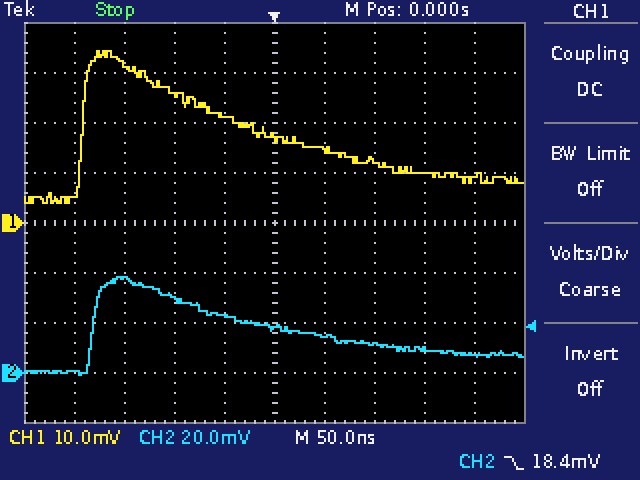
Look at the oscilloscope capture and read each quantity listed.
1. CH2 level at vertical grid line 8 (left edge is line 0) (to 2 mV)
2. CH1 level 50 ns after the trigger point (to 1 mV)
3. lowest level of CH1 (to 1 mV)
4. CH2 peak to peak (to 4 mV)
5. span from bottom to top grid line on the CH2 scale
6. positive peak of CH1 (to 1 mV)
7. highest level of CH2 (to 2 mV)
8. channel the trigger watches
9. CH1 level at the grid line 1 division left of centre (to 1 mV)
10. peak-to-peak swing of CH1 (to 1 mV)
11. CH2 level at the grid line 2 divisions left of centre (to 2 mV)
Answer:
10 mV
15 mV
4 mV
40 mV
160 mV
34 mV
38 mV
CH2
22 mV
30 mV
30 mV
